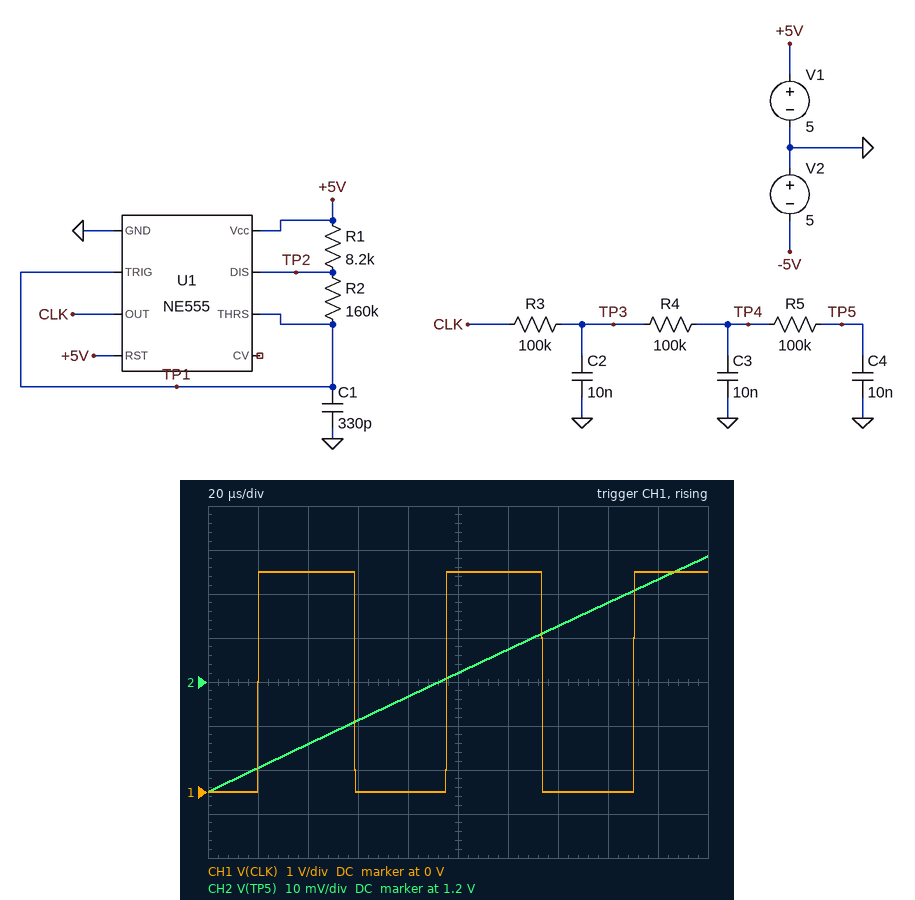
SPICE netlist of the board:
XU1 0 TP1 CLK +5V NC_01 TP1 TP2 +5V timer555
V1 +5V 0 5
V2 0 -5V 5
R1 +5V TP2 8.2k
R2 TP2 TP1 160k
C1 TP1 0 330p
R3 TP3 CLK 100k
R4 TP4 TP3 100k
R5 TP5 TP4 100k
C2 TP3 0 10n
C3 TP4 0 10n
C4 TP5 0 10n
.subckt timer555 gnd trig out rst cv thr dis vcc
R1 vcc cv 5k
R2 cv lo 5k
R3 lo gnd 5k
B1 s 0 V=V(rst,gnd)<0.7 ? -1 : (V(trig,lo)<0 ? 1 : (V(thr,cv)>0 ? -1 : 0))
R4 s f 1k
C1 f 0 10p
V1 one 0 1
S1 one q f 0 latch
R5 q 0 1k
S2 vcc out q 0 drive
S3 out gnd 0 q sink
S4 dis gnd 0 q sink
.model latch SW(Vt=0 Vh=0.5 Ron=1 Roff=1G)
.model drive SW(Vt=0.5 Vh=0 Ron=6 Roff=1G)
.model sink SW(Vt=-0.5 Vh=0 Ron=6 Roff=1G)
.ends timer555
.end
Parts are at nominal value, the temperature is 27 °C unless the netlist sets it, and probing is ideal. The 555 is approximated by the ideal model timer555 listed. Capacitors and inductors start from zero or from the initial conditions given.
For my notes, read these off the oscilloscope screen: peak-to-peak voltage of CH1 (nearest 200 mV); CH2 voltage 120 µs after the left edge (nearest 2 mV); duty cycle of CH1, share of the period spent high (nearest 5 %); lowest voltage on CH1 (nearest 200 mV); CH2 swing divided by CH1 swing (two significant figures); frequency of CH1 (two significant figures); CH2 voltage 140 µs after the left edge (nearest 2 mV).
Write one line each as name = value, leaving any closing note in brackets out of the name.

peak-to-peak voltage of CH1 = 5.0 V
CH2 voltage 120 µs after the left edge = 1.208 V
duty cycle of CH1, share of the period spent high = 50 %
lowest voltage on CH1 = 0 V
CH2 swing divided by CH1 swing = 0.011
frequency of CH1 = 13 kHz
CH2 voltage 140 µs after the left edge = 1.212 V
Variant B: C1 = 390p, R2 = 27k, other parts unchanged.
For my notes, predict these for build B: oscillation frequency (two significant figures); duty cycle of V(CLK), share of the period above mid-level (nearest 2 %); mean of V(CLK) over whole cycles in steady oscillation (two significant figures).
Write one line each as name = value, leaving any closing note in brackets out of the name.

oscillation frequency = 59 kHz
duty cycle of V(CLK), share of the period above mid-level = 56 %
mean of V(CLK) over whole cycles in steady oscillation = 2.8 V
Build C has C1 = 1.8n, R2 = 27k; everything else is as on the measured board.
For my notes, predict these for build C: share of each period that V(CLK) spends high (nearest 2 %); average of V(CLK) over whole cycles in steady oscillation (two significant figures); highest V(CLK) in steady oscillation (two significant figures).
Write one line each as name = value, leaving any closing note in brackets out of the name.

share of each period that V(CLK) spends high = 56 %
average of V(CLK) over whole cycles in steady oscillation = 2.8 V
highest V(CLK) in steady oscillation = 5.0 V
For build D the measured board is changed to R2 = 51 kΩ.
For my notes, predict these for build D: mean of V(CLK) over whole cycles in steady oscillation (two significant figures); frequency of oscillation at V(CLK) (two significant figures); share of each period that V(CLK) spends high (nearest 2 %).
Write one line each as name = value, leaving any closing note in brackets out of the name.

mean of V(CLK) over whole cycles in steady oscillation = 2.7 V
frequency of oscillation at V(CLK) = 40 kHz
share of each period that V(CLK) spends high = 54 %
